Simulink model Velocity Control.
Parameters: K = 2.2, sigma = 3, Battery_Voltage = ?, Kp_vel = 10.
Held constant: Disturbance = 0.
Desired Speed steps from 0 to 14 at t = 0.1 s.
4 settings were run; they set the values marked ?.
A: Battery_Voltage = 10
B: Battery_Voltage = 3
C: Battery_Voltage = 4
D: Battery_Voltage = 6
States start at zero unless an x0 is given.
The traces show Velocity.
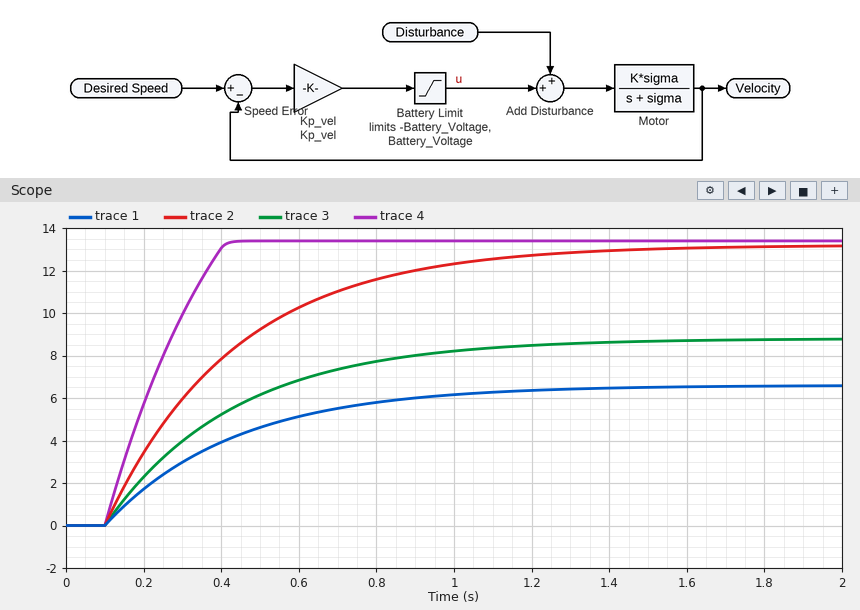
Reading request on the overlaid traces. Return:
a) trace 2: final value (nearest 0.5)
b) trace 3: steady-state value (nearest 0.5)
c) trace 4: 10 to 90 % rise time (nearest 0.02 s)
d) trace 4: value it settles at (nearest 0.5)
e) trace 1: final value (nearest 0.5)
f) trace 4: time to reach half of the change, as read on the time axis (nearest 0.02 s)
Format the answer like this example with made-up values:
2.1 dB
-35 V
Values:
13.0
9.0
0.24 s
13.5
6.5
0.22 s
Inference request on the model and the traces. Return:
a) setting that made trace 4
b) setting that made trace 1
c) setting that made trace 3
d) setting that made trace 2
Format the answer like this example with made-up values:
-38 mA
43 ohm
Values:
A
B
C
D
